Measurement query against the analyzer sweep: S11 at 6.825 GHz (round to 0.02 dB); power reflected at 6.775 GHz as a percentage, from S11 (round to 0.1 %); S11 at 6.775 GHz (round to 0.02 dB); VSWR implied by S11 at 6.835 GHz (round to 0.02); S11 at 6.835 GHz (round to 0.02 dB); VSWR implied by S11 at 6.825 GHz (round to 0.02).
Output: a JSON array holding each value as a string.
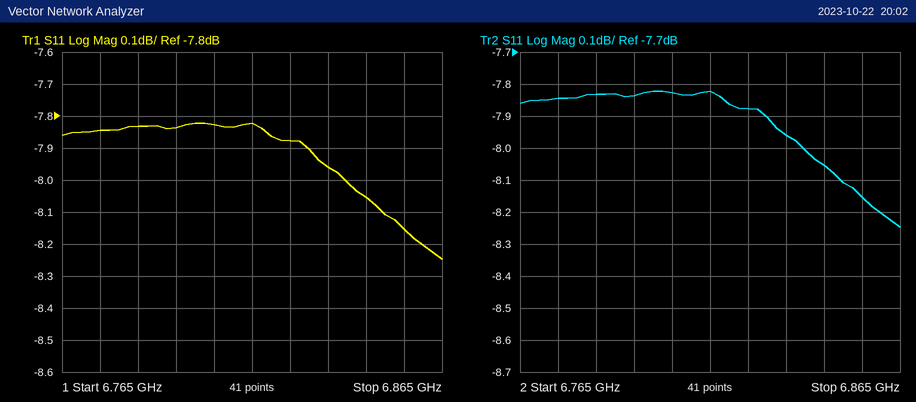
["-7.88 dB", "16.4 %", "-7.84 dB", "2.34", "-7.96 dB", "2.36"]
